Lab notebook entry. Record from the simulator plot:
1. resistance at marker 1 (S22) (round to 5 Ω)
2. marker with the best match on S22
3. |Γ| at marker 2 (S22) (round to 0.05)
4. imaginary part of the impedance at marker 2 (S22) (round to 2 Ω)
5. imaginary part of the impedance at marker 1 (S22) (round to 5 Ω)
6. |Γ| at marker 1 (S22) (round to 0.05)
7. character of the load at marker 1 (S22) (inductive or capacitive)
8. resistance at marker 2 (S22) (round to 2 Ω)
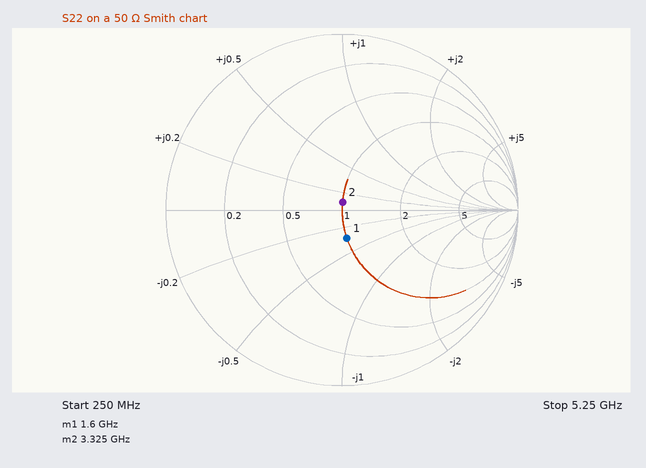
50 Ω
marker 2
0.05
+4 Ω
-15 Ω
0.15
capacitive
50 Ω
